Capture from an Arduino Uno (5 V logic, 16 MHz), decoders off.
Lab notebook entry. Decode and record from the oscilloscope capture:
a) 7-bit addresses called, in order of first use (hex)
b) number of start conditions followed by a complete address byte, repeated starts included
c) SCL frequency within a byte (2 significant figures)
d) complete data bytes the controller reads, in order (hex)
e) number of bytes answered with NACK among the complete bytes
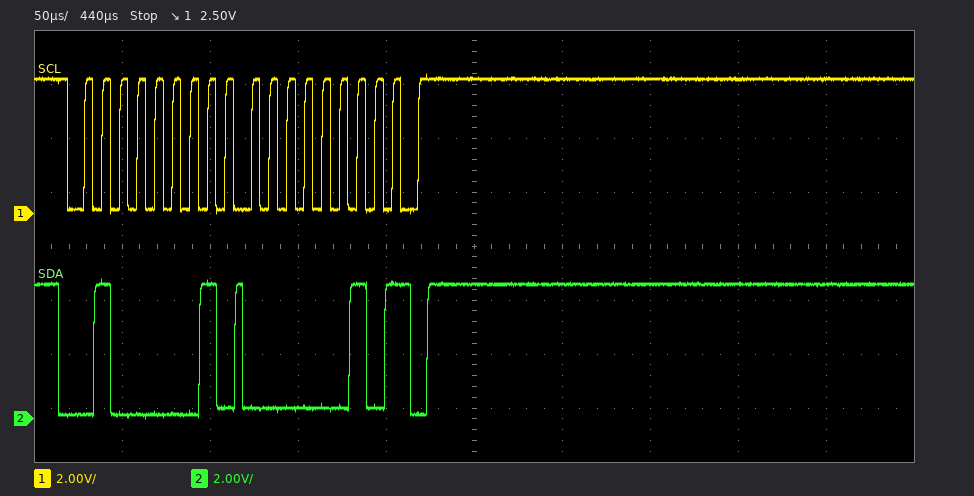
0x20
1
100 kHz
02
1
